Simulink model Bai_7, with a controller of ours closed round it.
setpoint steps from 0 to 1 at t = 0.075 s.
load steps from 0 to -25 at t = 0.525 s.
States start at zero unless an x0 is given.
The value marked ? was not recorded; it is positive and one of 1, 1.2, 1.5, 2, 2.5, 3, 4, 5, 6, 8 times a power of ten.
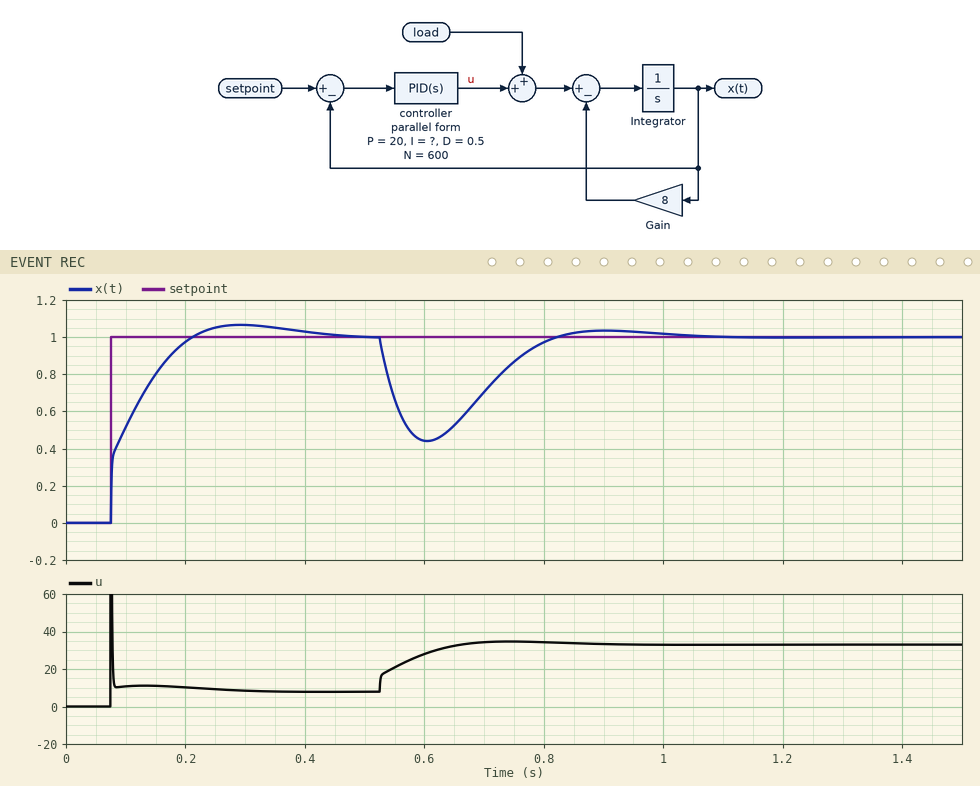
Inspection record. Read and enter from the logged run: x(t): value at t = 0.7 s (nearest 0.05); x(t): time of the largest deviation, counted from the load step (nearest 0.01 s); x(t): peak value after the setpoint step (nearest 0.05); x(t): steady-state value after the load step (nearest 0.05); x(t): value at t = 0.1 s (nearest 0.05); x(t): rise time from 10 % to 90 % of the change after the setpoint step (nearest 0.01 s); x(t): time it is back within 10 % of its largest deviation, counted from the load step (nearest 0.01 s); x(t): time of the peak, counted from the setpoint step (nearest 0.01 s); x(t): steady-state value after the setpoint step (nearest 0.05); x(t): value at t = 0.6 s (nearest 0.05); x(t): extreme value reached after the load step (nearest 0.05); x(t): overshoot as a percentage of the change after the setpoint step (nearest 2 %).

0.70
0.08 s
1.05
1.00
0.50
0.10 s
0.26 s
0.22 s
1.00
0.45
0.45
6 %
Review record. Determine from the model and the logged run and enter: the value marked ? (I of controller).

300
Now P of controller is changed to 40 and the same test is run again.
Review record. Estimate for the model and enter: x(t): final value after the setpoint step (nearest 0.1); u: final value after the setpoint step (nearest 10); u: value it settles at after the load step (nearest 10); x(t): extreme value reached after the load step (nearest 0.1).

1.0
10
30
0.6
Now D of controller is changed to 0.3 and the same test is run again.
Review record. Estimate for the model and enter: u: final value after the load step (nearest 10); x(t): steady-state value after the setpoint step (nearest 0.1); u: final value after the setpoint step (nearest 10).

30
1.0
10
